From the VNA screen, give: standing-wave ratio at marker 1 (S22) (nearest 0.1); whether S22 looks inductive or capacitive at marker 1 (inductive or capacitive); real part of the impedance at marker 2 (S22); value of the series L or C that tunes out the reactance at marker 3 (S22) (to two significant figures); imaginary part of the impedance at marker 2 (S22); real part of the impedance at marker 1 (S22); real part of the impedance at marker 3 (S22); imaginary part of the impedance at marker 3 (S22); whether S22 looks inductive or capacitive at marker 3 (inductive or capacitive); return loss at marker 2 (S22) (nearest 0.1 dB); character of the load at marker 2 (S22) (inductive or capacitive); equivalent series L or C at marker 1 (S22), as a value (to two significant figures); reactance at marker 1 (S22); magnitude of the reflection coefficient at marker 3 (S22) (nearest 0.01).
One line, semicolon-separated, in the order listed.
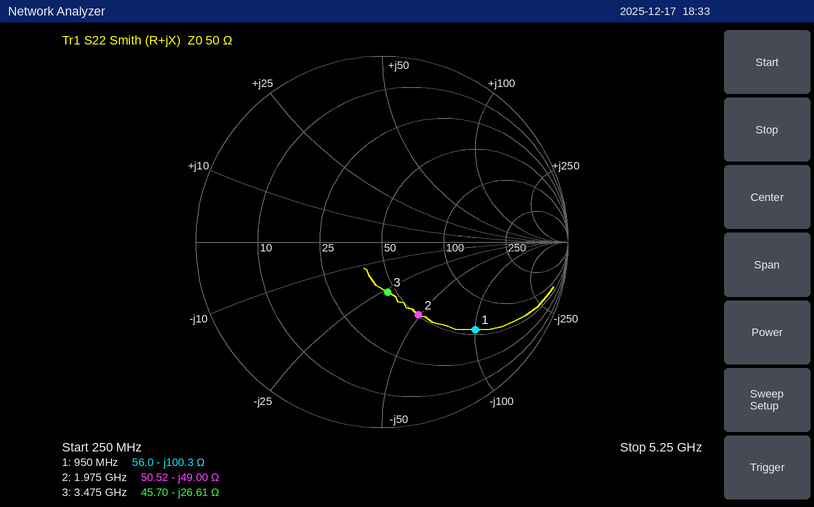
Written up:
5.4; capacitive; 50.52 Ω; 1.2 nH; -49.00 Ω; 56.0 Ω; 45.70 Ω; -26.61 Ω; capacitive; 7.2 dB; capacitive; 1.7 pF; -100.3 Ω; 0.27
